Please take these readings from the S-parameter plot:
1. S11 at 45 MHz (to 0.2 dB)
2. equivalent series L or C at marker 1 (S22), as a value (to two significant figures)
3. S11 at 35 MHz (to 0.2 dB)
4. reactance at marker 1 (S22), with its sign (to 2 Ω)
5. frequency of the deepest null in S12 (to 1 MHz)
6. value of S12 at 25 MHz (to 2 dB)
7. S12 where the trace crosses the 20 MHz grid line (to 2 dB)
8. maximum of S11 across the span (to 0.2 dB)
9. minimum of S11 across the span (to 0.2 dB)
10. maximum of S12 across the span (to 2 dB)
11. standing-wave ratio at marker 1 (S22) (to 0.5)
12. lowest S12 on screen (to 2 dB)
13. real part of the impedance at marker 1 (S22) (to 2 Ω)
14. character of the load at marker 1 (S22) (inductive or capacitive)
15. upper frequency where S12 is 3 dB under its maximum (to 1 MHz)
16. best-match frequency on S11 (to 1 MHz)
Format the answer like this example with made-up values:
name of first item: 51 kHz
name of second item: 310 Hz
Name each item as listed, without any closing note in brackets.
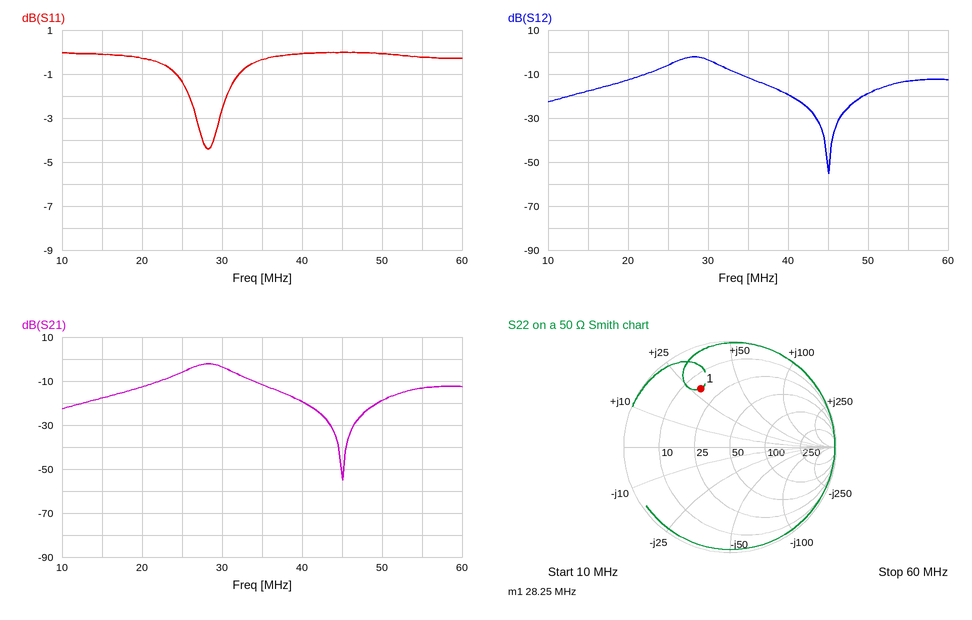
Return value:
S11 at 45 MHz: 0.0 dB
equivalent series L or C at marker 1 (S22), as a value: 160 nH
S11 at 35 MHz: -0.4 dB
reactance at marker 1 (S22), with its sign: +28 Ω
frequency of the deepest null in S12: 45 MHz
value of S12 at 25 MHz: -6 dB
S12 where the trace crosses the 20 MHz grid line: -12 dB
maximum of S11 across the span: 0.0 dB
minimum of S11 across the span: -4.4 dB
maximum of S12 across the span: -2 dB
standing-wave ratio at marker 1 (S22): 4.0
lowest S12 on screen: -56 dB
real part of the impedance at marker 1 (S22): 16 Ω
character of the load at marker 1 (S22): inductive
upper frequency where S12 is 3 dB under its maximum: 31 MHz
best-match frequency on S11: 28 MHz
